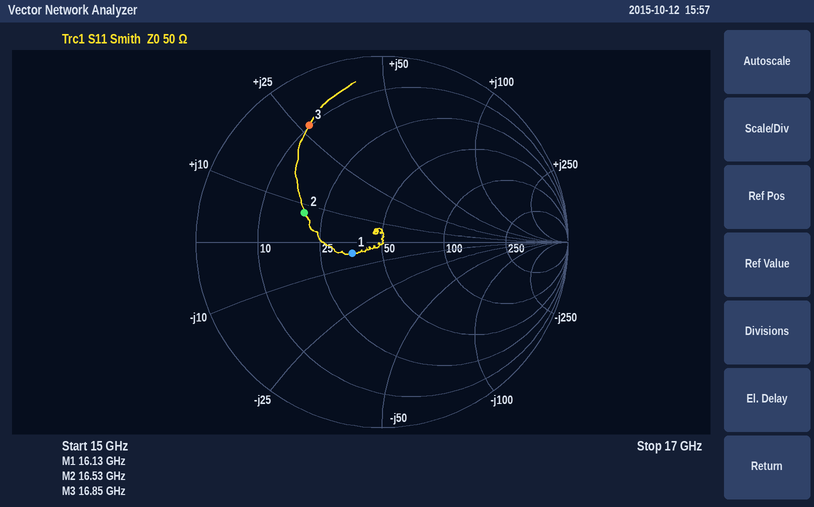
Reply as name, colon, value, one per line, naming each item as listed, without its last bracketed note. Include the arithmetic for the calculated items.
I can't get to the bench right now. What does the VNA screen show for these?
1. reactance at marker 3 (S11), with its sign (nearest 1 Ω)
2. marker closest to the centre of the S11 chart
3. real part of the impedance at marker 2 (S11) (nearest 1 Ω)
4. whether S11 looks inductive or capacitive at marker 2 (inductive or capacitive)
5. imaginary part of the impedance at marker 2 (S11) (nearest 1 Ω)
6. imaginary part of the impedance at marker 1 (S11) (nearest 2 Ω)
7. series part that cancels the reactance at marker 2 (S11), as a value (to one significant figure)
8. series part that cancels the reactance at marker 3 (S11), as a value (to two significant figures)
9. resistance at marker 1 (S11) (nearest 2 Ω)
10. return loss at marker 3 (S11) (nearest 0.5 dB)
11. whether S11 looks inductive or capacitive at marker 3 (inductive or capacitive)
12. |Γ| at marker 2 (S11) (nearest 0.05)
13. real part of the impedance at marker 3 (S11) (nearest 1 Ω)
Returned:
reactance at marker 3 (S11), with its sign: +27 Ω
marker closest to the centre of the S11 chart: marker 1
real part of the impedance at marker 2 (S11): 20 Ω
whether S11 looks inductive or capacitive at marker 2: inductive
imaginary part of the impedance at marker 2 (S11): +8 Ω
imaginary part of the impedance at marker 1 (S11): -4 Ω
series part that cancels the reactance at marker 2 (S11), as a value: C = 1/(2π × 16.53 GHz × 8 Ω) ≈ 1 pF
series part that cancels the reactance at marker 3 (S11), as a value: C = 1/(2π × 16.85 GHz × 27 Ω) ≈ 350 fF
resistance at marker 1 (S11): 36 Ω
return loss at marker 3 (S11): 2.5 dB
whether S11 looks inductive or capacitive at marker 3: inductive
|Γ| at marker 2 (S11): 0.45
real part of the impedance at marker 3 (S11): 10 Ω
